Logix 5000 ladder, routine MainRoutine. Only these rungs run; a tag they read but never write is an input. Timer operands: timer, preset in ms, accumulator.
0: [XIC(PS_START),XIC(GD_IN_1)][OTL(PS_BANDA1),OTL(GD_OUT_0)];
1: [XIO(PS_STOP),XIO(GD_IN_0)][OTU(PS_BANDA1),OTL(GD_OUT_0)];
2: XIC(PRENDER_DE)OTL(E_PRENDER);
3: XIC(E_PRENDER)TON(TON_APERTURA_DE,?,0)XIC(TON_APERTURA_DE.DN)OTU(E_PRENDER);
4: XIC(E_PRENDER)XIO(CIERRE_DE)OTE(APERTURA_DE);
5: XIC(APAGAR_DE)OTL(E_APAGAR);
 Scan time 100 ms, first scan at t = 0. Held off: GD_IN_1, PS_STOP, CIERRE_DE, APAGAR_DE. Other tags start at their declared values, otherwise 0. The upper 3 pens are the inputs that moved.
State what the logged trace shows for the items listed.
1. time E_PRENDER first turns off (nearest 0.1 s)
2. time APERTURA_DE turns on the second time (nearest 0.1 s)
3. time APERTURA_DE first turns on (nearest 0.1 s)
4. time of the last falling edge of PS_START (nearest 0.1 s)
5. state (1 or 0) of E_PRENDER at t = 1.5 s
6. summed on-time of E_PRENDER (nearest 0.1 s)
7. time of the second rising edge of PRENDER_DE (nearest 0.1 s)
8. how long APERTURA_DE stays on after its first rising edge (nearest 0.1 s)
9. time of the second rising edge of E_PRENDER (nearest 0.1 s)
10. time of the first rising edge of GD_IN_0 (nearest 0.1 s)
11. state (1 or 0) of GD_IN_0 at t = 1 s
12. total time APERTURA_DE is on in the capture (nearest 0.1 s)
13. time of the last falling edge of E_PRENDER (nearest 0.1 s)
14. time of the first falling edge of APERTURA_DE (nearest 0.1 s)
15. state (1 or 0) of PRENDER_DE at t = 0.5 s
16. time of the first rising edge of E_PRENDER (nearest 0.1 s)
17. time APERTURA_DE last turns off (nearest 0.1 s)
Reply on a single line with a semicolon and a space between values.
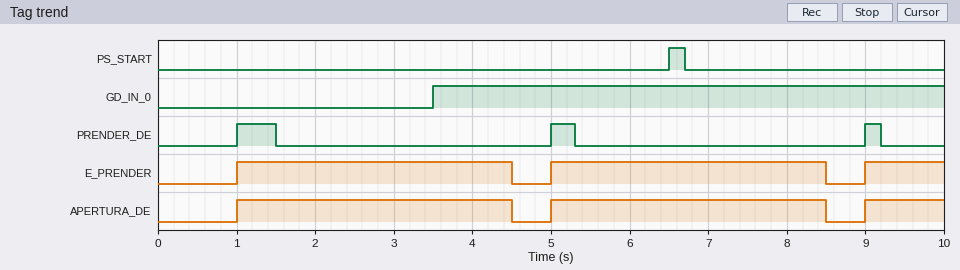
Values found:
4.5 s; 5.0 s; 1.0 s; 6.7 s; 1; 8.0 s; 5.0 s; 3.5 s; 5.0 s; 3.5 s; 0; 8.0 s; 8.5 s; 4.5 s; 0; 1.0 s; 8.5 s
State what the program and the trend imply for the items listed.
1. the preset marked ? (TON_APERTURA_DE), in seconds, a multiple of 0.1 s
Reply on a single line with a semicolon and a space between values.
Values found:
3.5 s
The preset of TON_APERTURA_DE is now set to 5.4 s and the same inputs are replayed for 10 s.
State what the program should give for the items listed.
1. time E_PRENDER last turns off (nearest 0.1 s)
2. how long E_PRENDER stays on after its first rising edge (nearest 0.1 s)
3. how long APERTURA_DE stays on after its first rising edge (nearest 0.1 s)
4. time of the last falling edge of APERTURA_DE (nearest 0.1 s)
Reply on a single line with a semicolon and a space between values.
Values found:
6.4 s; 5.4 s; 5.4 s; 6.4 s
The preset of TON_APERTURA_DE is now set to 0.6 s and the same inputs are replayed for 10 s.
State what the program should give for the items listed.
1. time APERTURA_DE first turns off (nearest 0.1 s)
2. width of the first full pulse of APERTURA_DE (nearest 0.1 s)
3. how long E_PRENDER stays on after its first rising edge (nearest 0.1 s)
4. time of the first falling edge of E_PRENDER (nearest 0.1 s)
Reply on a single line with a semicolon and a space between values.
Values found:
1.6 s; 0.6 s; 0.6 s; 1.6 s
